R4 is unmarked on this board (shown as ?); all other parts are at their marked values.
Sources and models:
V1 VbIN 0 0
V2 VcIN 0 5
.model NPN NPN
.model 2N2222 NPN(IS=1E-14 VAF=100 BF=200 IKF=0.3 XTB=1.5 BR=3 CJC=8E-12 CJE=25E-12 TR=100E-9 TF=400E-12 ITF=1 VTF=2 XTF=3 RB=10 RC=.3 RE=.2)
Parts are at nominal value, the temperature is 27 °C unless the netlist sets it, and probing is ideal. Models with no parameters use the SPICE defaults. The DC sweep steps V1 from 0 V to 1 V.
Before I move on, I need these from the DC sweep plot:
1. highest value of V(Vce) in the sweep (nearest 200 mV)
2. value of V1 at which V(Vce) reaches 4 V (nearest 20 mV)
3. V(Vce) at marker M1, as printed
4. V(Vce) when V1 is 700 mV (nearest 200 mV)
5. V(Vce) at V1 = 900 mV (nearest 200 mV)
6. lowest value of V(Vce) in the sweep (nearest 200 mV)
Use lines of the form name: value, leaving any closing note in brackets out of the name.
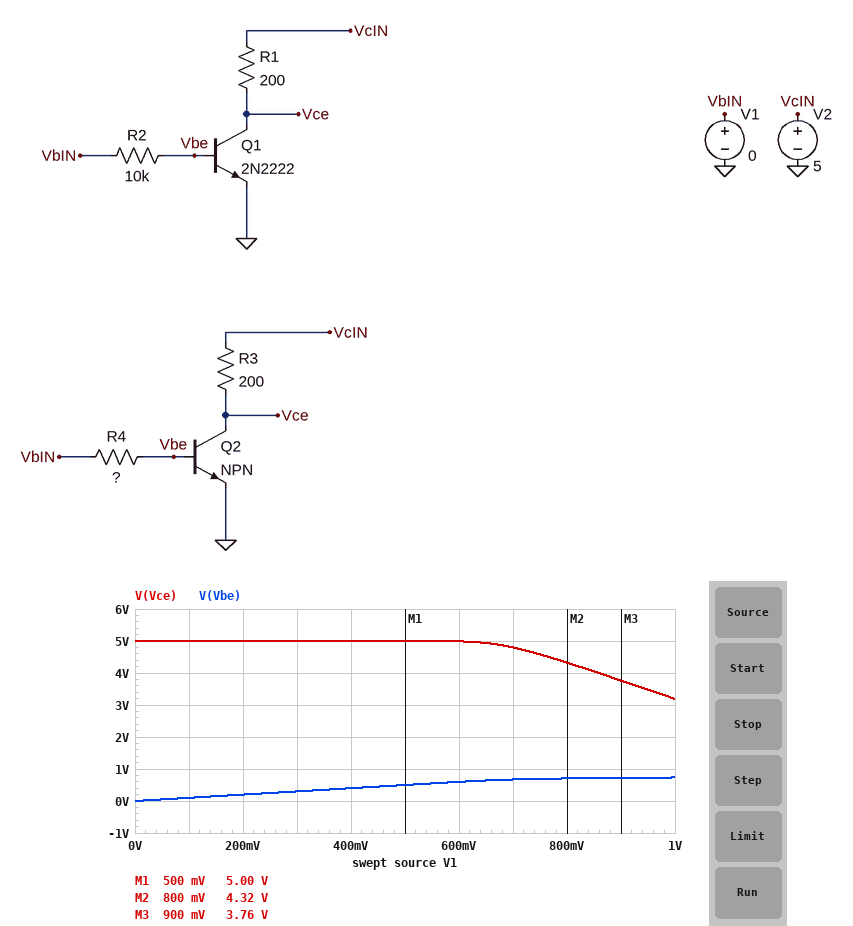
highest value of V(Vce) in the sweep: 5.0 V
value of V1 at which V(Vce) reaches 4 V: 860 mV
V(Vce) at marker M1, as printed: 5.00 V
V(Vce) when V1 is 700 mV: 4.8 V
V(Vce) at V1 = 900 mV: 3.8 V
lowest value of V(Vce) in the sweep: 3.2 V
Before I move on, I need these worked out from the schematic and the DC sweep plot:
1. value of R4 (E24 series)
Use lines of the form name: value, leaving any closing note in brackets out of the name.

value of R4: 3.9 kΩ
